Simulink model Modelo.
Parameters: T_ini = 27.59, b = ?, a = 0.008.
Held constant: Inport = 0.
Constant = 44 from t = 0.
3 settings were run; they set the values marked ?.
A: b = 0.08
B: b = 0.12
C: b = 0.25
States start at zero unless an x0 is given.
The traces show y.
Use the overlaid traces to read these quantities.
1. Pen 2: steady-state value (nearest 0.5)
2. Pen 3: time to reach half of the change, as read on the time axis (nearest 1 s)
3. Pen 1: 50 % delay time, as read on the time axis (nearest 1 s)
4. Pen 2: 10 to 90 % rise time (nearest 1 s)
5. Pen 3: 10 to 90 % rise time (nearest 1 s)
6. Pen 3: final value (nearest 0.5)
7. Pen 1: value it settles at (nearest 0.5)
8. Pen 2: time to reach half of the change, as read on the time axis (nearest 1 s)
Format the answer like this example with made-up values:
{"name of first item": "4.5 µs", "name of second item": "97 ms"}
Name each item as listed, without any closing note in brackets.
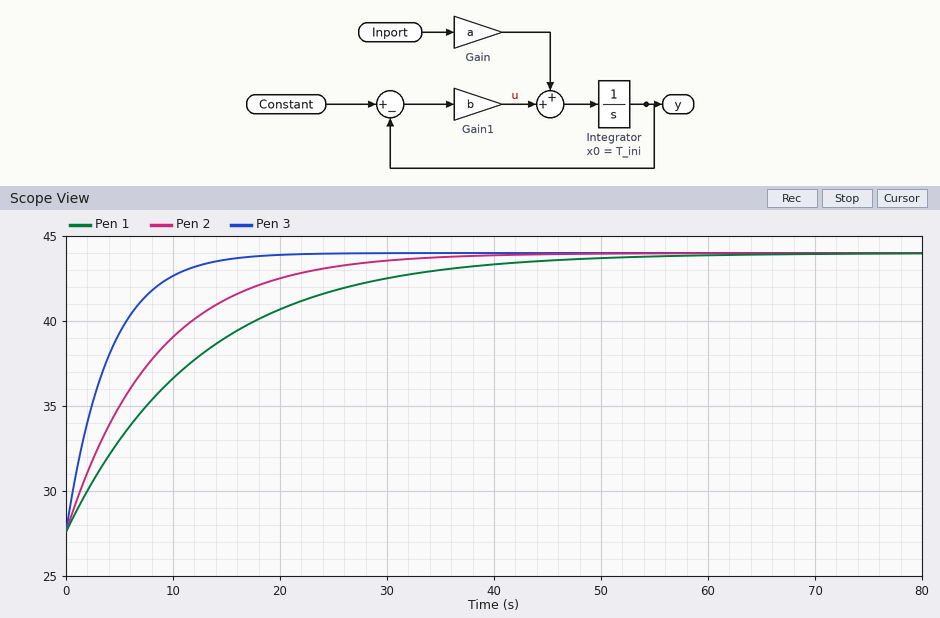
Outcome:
{"Pen 2: steady-state value": "44.0", "Pen 3: time to reach half of the change, as read on the time axis": "3 s", "Pen 1: 50 % delay time, as read on the time axis": "9 s", "Pen 2: 10 to 90 % rise time": "18 s", "Pen 3: 10 to 90 % rise time": "9 s", "Pen 3: final value": "44.0", "Pen 1: value it settles at": "44.0", "Pen 2: time to reach half of the change, as read on the time axis": "6 s"}
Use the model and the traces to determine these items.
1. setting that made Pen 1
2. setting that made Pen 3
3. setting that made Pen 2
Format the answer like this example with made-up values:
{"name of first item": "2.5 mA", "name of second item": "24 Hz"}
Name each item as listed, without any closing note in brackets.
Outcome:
{"setting that made Pen 1": "A", "setting that made Pen 3": "C", "setting that made Pen 2": "B"}
